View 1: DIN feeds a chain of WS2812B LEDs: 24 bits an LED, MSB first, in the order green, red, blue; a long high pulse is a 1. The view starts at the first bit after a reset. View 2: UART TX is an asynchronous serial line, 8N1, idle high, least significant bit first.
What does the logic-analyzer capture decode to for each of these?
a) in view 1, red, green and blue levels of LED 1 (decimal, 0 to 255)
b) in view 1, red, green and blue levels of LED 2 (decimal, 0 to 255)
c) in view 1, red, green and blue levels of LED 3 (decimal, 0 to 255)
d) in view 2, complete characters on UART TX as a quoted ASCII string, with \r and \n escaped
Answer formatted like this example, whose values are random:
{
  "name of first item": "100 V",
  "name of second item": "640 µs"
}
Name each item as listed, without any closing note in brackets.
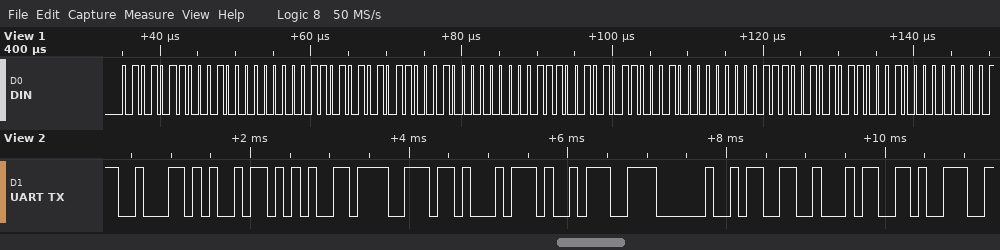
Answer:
{
  "in view 1, red, green and blue levels of LED 1": "32, 86, 13",
  "in view 1, red, green and blue levels of LED 2": "32, 86, 14",
  "in view 1, red, green and blue levels of LED 3": "32, 86, 14",
  "in view 2, complete characters on UART TX as a quoted ASCII string, with \\r and \\n escaped": "\"bient: 349\""
}
